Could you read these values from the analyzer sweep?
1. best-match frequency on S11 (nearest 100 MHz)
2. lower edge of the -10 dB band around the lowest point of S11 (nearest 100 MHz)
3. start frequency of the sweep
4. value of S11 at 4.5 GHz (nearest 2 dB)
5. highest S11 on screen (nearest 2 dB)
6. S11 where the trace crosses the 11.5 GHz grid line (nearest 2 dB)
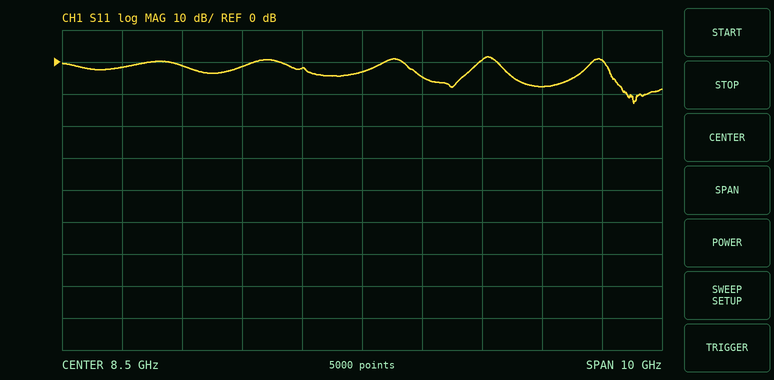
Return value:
13.0 GHz
12.9 GHz
3.5 GHz
-2 dB
2 dB
-8 dB
